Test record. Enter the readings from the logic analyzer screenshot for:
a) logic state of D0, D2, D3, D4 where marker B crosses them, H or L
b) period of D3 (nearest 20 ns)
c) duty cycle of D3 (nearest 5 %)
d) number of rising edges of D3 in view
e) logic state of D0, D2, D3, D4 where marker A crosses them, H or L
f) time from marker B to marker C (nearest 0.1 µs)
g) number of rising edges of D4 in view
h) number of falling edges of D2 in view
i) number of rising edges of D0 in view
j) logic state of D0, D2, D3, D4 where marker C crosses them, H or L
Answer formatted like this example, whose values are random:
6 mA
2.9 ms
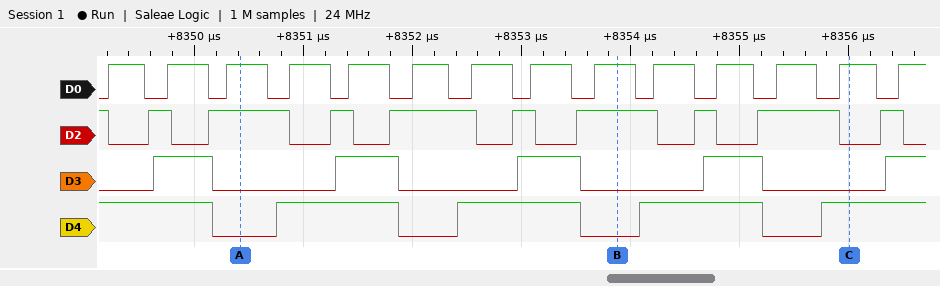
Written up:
D0=H, D2=H, D3=L, D4=L
1680 ns
35 %
5
D0=H, D2=H, D3=L, D4=L
2.1 µs
4
10
14
D0=H, D2=L, D3=L, D4=H
